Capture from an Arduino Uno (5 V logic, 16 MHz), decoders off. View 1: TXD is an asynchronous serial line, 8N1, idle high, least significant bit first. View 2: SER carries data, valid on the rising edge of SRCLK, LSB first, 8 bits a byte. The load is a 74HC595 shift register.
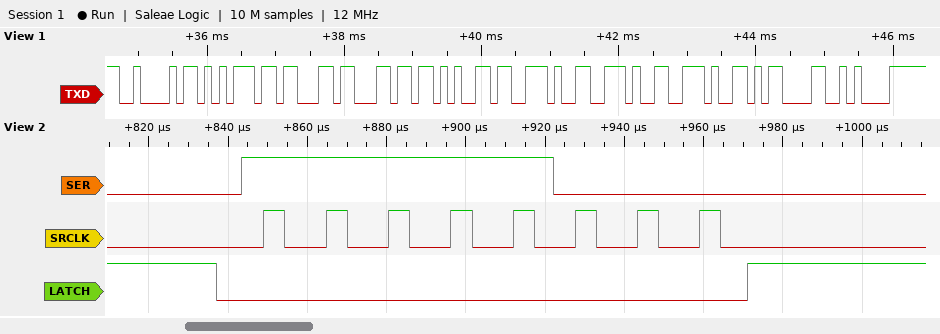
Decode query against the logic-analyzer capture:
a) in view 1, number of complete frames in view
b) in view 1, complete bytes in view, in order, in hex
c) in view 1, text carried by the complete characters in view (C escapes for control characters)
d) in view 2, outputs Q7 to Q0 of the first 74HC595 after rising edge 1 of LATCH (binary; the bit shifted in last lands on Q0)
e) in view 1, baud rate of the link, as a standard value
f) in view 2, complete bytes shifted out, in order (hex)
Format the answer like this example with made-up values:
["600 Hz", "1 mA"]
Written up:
["10", "42 75 63 6C 65 2E 2E 2E 0D 0A", "\"Bucle...\\r\\n\"", "11111000", "9600 baud", "1F"]
